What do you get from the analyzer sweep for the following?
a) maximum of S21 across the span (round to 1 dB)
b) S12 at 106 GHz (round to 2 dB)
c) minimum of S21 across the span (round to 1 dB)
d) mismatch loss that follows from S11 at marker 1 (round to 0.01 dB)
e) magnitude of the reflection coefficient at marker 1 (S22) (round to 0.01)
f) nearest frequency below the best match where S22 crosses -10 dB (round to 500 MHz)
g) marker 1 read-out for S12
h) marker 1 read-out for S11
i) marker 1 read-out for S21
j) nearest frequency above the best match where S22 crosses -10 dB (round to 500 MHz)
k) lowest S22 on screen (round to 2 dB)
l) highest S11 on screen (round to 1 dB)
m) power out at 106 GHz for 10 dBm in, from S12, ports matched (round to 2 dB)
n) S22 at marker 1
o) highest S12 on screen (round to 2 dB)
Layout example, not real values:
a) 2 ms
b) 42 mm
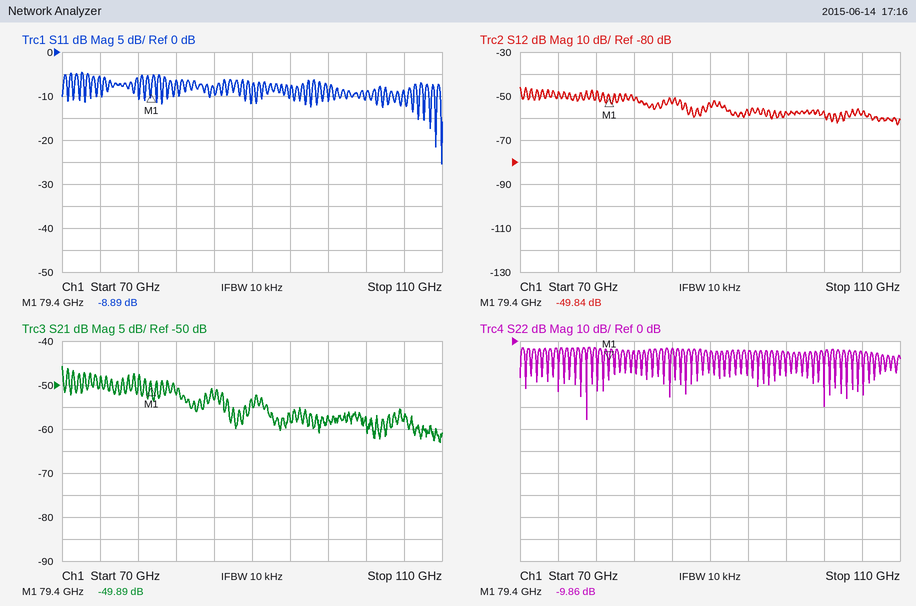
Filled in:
a) -46 dB
b) -58 dB
c) -63 dB
d) 0.60 dB
e) 0.32
f) 77.0 GHz
g) -49.84 dB
h) -8.89 dB
i) -49.89 dB
j) 77.0 GHz
k) -36 dB
l) -5 dB
m) -48 dBm
n) -9.86 dB
o) -46 dB
